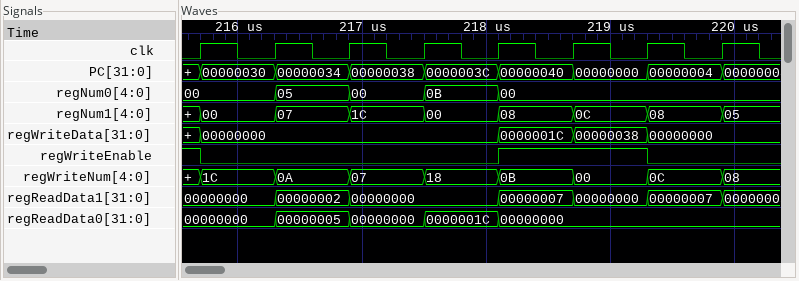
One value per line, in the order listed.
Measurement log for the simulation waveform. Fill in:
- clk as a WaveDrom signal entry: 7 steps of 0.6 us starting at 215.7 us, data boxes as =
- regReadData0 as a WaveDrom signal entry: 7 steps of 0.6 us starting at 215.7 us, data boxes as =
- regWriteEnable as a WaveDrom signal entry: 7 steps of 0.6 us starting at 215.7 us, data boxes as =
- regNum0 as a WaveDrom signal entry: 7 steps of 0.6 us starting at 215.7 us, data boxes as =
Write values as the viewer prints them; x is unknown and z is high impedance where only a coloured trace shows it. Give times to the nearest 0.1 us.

{name: 'clk', wave: 'p......'}
{name: 'regReadData0', wave: '=====..', data: '00000000 00000005 00000000 0000001C 00000000'}
{name: 'regWriteEnable', wave: '0...1.0'}
{name: 'regNum0', wave: '=====..', data: '00 05 00 0B 00'}
